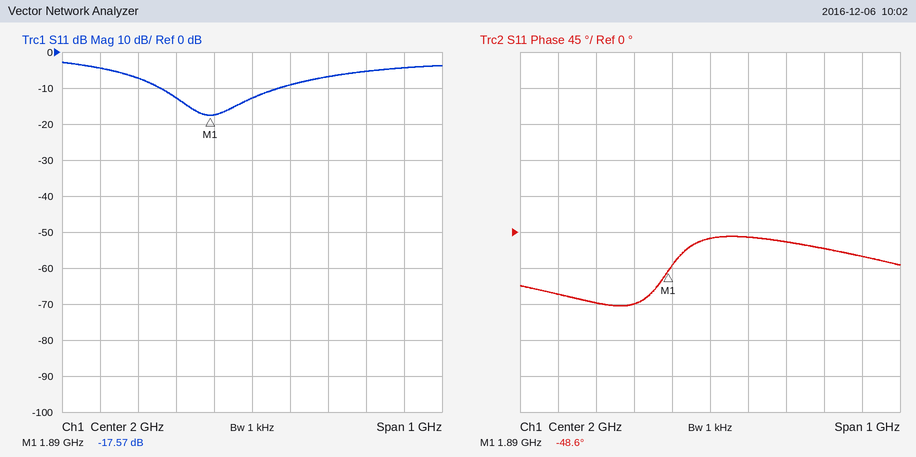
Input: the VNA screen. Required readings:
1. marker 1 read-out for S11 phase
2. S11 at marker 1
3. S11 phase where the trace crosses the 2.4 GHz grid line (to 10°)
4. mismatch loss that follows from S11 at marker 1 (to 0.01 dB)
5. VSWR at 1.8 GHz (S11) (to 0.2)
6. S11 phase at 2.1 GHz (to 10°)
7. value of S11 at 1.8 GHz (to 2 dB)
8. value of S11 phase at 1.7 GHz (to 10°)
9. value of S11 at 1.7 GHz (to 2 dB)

-48.6°
-17.57 dB
-30°
0.08 dB
1.6
-10°
-12 dB
-90°
-8 dB
